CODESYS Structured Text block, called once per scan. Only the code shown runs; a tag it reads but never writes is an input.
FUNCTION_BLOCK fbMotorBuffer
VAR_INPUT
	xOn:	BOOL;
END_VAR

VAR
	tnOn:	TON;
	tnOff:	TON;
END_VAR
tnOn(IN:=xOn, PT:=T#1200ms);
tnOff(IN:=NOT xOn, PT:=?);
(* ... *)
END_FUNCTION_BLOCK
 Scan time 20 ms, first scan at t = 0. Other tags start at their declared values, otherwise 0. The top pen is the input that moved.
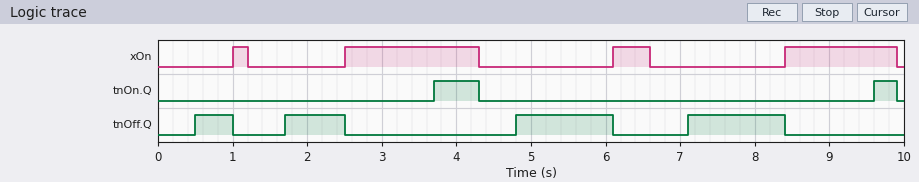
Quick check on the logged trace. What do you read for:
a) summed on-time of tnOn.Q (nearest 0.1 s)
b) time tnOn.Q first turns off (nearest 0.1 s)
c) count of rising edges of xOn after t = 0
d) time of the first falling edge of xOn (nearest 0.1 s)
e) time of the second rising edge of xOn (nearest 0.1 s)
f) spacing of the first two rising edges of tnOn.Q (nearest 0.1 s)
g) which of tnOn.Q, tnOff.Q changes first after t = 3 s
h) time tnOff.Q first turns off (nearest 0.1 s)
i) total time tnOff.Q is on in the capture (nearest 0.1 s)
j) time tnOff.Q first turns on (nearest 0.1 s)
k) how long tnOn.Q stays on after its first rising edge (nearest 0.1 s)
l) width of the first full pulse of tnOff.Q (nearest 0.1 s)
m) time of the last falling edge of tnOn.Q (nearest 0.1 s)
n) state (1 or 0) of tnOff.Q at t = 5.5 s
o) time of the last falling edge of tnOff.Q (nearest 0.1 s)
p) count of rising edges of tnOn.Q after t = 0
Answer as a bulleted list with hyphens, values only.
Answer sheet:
- 0.9 s
- 4.3 s
- 4
- 1.2 s
- 2.5 s
- 5.9 s
- tnOn.Q
- 1.0 s
- 3.9 s
- 0.5 s
- 0.6 s
- 0.5 s
- 9.9 s
- 1
- 8.4 s
- 2
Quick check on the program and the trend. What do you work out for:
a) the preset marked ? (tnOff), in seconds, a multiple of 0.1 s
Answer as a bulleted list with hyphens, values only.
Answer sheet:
- 0.5 s
